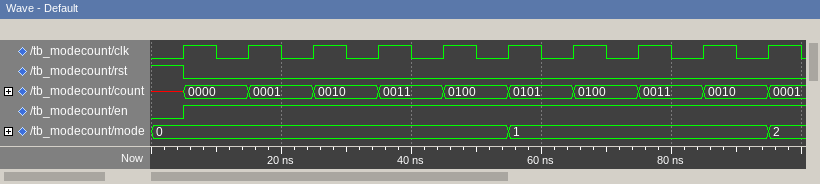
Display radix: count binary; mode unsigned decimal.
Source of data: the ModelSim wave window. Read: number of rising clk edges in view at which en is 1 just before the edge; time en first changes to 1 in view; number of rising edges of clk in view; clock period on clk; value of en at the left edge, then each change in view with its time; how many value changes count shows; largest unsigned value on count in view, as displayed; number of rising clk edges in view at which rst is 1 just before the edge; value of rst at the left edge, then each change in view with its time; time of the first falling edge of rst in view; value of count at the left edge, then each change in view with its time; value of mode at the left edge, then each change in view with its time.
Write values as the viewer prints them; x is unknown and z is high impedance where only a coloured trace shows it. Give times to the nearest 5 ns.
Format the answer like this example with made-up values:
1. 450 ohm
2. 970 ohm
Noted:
1. 9
2. 5 ns
3. 10
4. 10 ns
5. 0, 1 at 5 ns
6. 10
7. 0101
8. 1
9. 1, 0 at 5 ns
10. 5 ns
11. x, 0000 at 5 ns, 0001 at 15 ns, 0010 at 25 ns, 0011 at 35 ns, 0100 at 45 ns, 0101 at 55 ns, 0100 at 65 ns, 0011 at 75 ns, 0010 at 85 ns, 0001 at 95 ns
12. 0, 1 at 55 ns, 2 at 95 ns
